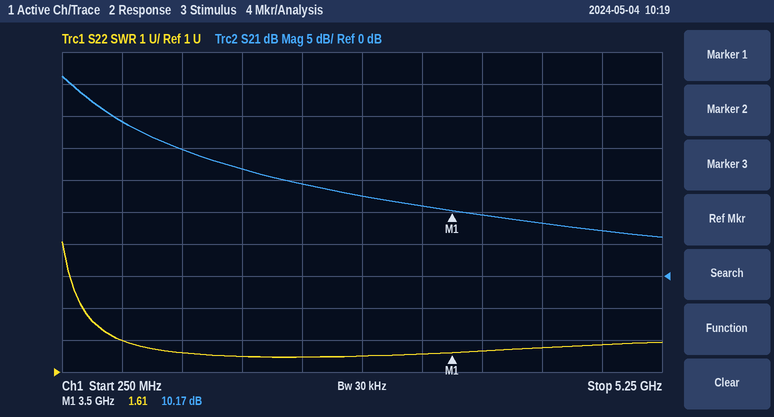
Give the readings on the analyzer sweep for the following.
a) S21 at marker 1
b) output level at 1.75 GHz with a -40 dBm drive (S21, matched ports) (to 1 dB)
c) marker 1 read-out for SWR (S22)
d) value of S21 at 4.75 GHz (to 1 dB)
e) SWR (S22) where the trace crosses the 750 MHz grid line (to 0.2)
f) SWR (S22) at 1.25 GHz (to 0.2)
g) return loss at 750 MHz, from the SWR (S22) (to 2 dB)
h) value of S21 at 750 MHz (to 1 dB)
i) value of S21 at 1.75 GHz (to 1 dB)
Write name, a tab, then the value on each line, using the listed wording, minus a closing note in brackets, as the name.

S21 at marker 1	10.17 dB
output level at 1.75 GHz with a -40 dBm drive (S21, matched ports)	-23 dBm
marker 1 read-out for SWR	1.61
value of S21 at 4.75 GHz	7 dB
SWR (S22) where the trace crosses the 750 MHz grid line	2.0
SWR (S22) at 1.25 GHz	1.6
return loss at 750 MHz, from the SWR (S22)	10 dB
value of S21 at 750 MHz	24 dB
value of S21 at 1.75 GHz	17 dB
